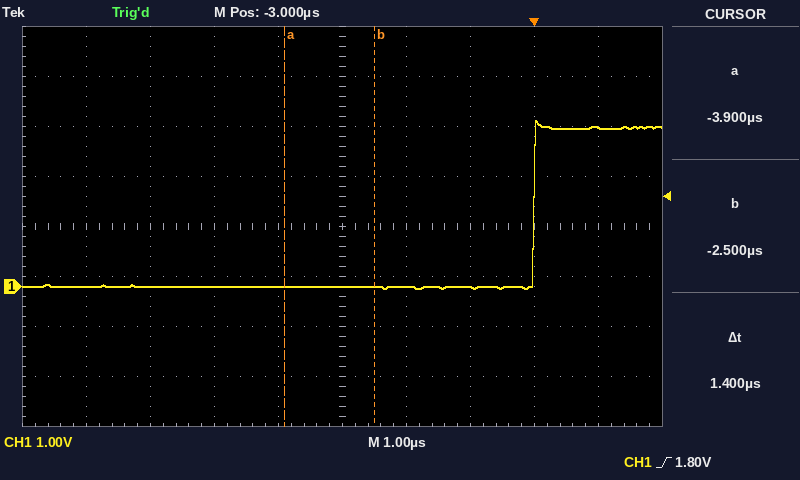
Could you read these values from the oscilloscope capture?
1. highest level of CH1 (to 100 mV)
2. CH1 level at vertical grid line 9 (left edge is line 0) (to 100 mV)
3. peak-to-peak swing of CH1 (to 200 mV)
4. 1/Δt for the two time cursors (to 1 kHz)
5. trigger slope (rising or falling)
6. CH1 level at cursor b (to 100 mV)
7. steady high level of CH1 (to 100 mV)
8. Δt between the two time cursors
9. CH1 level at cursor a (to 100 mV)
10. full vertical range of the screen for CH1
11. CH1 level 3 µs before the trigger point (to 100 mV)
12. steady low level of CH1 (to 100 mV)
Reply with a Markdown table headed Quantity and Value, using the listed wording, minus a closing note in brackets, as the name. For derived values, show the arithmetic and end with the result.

| Quantity | Value |
|---|---|
| highest level of CH1 | 3.3 V |
| CH1 level at vertical grid line 9 (left edge is line 0) | 3.2 V |
| peak-to-peak swing of CH1 | 3.4 V |
| 1/Δt for the two time cursors | 1 / 1.4 µs ≈ 714 kHz |
| trigger slope | rising |
| CH1 level at cursor b | 0.0 V |
| steady high level of CH1 | 3.2 V |
| Δt between the two time cursors | 1.4 µs |
| CH1 level at cursor a | 0.0 V |
| full vertical range of the screen for CH1 | 8 V |
| CH1 level 3 µs before the trigger point | 0.0 V |
| steady low level of CH1 | 0.0 V |
